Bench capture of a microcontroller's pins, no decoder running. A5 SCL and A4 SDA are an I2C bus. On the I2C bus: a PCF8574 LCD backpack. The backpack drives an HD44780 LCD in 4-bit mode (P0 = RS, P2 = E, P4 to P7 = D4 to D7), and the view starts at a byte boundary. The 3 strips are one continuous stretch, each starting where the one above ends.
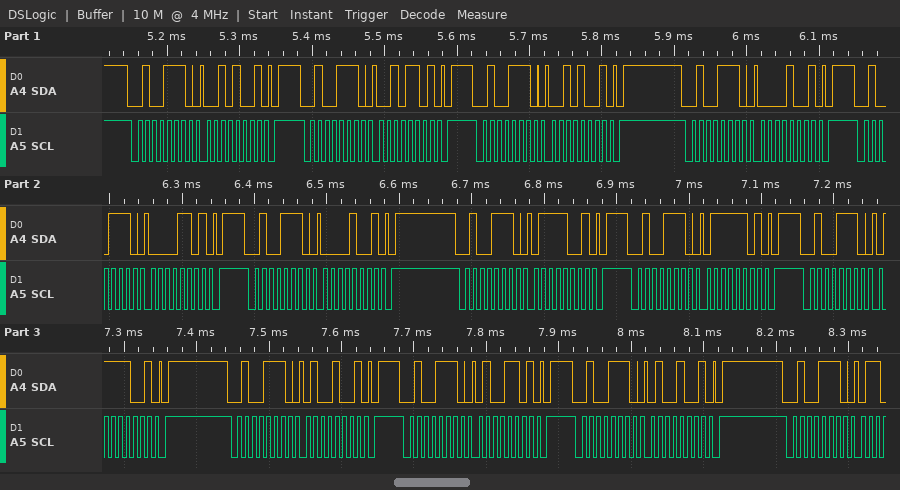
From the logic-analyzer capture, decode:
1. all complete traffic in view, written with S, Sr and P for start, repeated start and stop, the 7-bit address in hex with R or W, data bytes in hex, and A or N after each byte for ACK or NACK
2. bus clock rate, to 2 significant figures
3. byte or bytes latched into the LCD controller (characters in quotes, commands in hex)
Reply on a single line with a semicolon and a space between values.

S 27W A 29 A P S 27W A 2D A P S 27W A 29 A P S 27W A 09 A P S 27W A 0D A P S 27W A 09 A P S 27W A 79 A P S 27W A 7D A P S 27W A 79 A P S 27W A 49 A P S 27W A 4D A P S 27W A 49 A P S 27W A; 100 kHz; ' ' 't'
